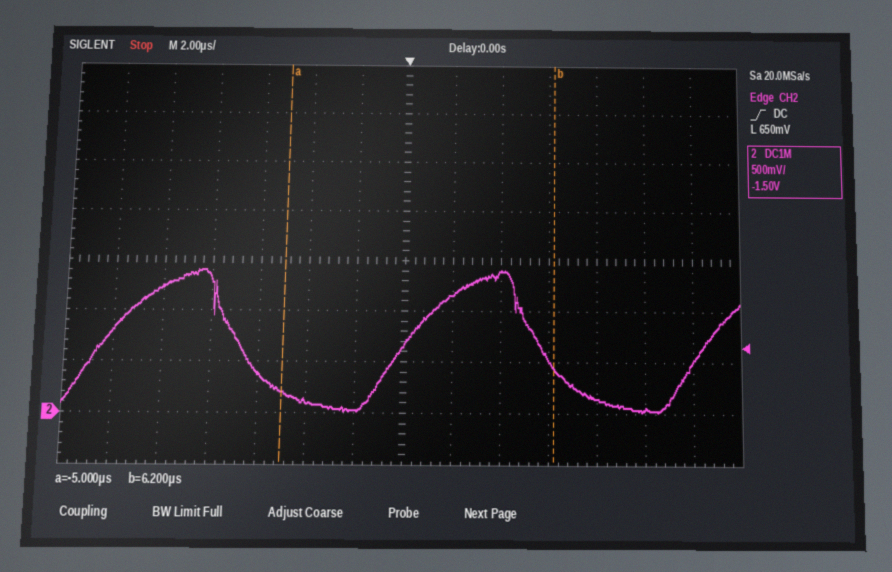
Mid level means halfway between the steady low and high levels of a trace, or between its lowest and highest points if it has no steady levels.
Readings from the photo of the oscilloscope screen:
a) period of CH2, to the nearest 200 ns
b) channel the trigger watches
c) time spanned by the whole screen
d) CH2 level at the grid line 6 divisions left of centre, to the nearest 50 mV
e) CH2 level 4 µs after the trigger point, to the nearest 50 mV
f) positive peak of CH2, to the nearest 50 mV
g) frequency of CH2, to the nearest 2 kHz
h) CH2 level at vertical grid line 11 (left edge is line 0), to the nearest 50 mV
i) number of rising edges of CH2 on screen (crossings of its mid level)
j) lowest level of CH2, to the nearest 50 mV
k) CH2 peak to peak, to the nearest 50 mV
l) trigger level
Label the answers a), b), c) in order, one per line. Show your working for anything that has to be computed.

a) 12.4 µs
b) CH2
c) 28 µs
d) 800 mV
e) 1.40 V
f) 1.40 V
g) 1 / 12.4 µs ≈ 80.6 kHz, so 80 kHz to the nearest 2 kHz
h) 150 mV
i) 3
j) 0 mV
k) 1.40 V − (0 mV) = 1.40 V
l) 650 mV
